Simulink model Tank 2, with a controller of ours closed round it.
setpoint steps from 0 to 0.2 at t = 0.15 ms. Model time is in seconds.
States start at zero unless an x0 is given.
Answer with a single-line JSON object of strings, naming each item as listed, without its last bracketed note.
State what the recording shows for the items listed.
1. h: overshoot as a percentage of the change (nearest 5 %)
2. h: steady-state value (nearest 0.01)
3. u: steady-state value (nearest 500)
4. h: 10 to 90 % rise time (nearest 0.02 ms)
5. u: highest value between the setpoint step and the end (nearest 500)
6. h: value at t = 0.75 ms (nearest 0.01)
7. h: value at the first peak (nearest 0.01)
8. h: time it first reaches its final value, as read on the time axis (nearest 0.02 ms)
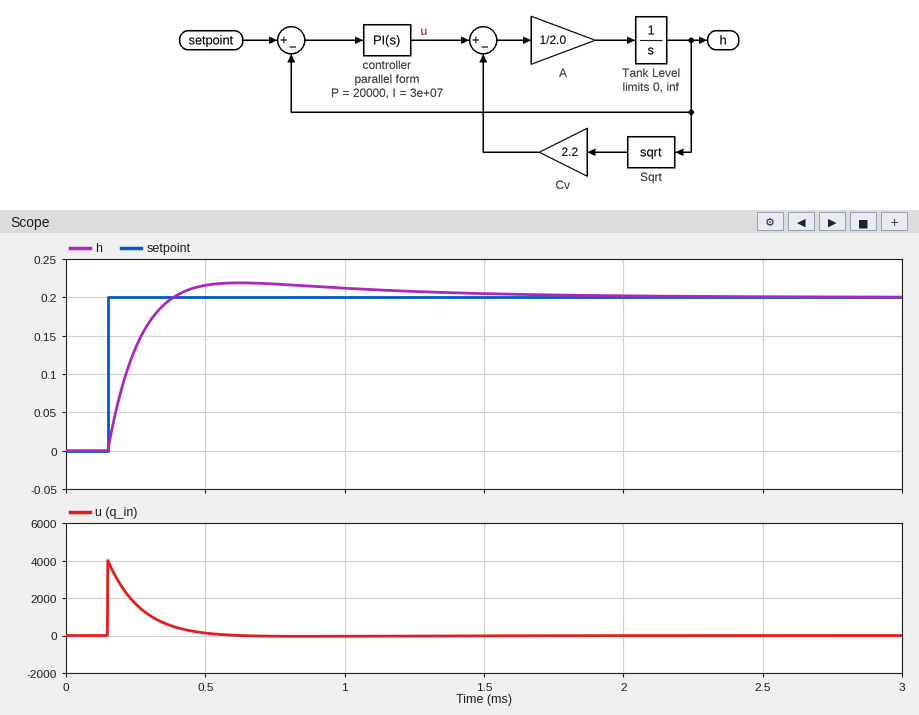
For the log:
{"h: overshoot as a percentage of the change": "10 %", "h: steady-state value": "0.20", "u: steady-state value": "0", "h: 10 to 90 % rise time": "0.16 ms", "u: highest value between the setpoint step and the end": "4000", "h: value at t = 0.75 ms": "0.22", "h: value at the first peak": "0.22", "h: time it first reaches its final value, as read on the time axis": "0.38 ms"}
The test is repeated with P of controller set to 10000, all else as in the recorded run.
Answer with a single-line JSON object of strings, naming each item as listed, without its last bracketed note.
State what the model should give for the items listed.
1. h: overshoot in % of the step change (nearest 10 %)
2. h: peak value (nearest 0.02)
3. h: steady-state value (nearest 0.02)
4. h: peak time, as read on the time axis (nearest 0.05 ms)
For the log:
{"h: overshoot in % of the step change": "20 %", "h: peak value": "0.24", "h: steady-state value": "0.20", "h: peak time, as read on the time axis": "0.75 ms"}
